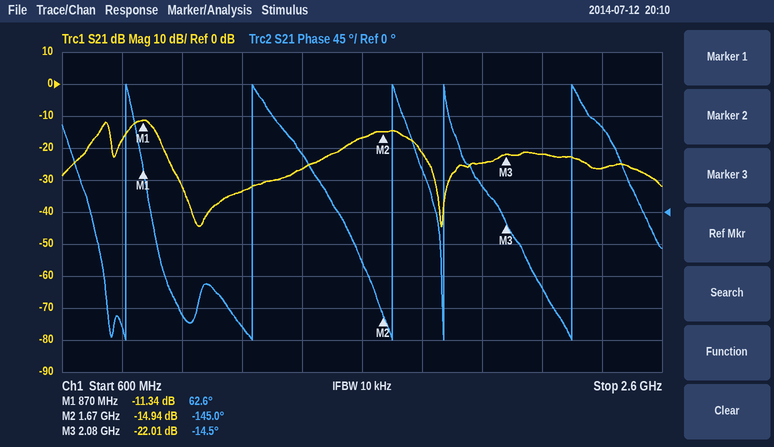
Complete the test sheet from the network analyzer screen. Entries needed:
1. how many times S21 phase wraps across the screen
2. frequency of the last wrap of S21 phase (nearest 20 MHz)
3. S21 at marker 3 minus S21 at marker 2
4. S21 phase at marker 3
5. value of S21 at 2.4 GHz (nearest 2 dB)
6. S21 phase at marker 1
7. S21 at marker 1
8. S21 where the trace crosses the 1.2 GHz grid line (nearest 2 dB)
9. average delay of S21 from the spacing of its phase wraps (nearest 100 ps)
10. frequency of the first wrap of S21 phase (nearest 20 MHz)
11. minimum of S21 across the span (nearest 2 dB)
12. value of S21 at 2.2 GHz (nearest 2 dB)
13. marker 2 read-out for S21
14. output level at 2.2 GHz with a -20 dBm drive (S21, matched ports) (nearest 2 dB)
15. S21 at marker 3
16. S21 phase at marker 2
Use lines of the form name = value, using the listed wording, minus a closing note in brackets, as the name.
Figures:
how many times S21 phase wraps across the screen = 5
frequency of the last wrap of S21 phase = 2.30 GHz
S21 at marker 3 minus S21 at marker 2 = -7.07 dB
S21 phase at marker 3 = -14.5°
value of S21 at 2.4 GHz = -26 dB
S21 phase at marker 1 = 62.6°
S21 at marker 1 = -11.34 dB
S21 where the trace crosses the 1.2 GHz grid line = -34 dB
average delay of S21 from the spacing of its phase wraps = 2.7 ns
frequency of the first wrap of S21 phase = 820 MHz
minimum of S21 across the span = -44 dB
value of S21 at 2.2 GHz = -22 dB
marker 2 read-out for S21 = -14.94 dB
output level at 2.2 GHz with a -20 dBm drive (S21, matched ports) = -42 dBm
S21 at marker 3 = -22.01 dB
S21 phase at marker 2 = -145.0°
